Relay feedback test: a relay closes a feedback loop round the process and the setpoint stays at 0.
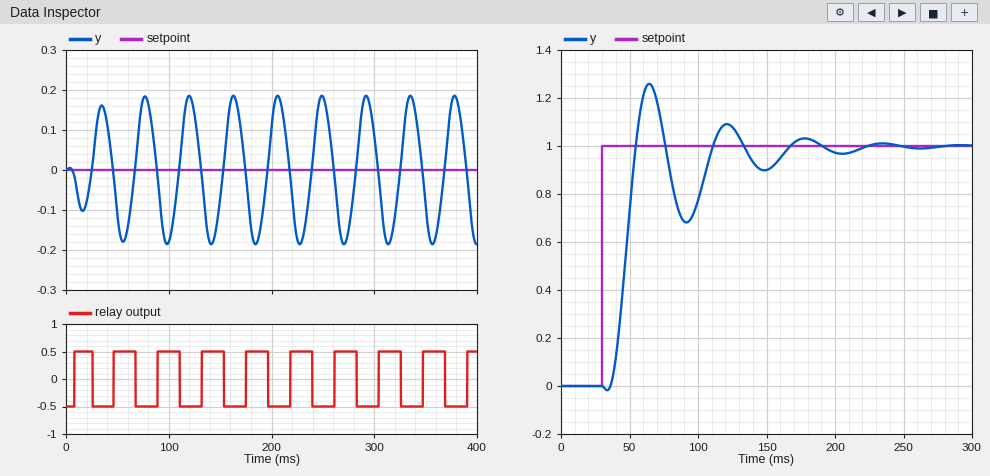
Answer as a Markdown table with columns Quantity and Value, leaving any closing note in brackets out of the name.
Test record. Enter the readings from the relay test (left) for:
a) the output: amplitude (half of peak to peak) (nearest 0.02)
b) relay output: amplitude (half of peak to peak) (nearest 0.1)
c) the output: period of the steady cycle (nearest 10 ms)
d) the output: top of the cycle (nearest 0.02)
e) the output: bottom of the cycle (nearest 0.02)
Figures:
| Quantity | Value |
|---|---|
| the output: amplitude (half of peak to peak) | 0.18 |
| relay output: amplitude (half of peak to peak) | 0.5 |
| the output: period of the steady cycle | 40 ms |
| the output: top of the cycle | 0.18 |
| the output: bottom of the cycle | -0.18 |
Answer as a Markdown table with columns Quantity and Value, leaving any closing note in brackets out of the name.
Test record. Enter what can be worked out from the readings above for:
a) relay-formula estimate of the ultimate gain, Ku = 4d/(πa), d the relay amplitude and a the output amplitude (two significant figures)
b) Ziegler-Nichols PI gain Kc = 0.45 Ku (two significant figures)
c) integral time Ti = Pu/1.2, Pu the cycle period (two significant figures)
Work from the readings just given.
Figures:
| Quantity | Value |
|---|---|
| relay-formula estimate of the ultimate gain, Ku = 4d/(πa), d the relay amplitude and a the output amplitude | 3.5 |
| Ziegler-Nichols PI gain Kc = 0.45 Ku | 1.6 |
| integral time Ti = Pu/1.2, Pu the cycle period | 33 ms |
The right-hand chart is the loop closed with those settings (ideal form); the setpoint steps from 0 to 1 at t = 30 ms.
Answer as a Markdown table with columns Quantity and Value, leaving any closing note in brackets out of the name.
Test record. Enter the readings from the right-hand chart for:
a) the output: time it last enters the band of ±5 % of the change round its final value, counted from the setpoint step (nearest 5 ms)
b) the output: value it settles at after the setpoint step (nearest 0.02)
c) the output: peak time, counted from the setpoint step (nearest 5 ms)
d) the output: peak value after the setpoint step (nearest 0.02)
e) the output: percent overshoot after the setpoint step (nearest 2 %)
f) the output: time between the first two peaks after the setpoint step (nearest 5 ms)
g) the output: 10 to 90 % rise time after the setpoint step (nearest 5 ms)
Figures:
| Quantity | Value |
|---|---|
| the output: time it last enters the band of ±5 % of the change round its final value, counted from the setpoint step | 130 ms |
| the output: value it settles at after the setpoint step | 1.00 |
| the output: peak time, counted from the setpoint step | 35 ms |
| the output: peak value after the setpoint step | 1.26 |
| the output: percent overshoot after the setpoint step | 26 % |
| the output: time between the first two peaks after the setpoint step | 55 ms |
| the output: 10 to 90 % rise time after the setpoint step | 15 ms |
